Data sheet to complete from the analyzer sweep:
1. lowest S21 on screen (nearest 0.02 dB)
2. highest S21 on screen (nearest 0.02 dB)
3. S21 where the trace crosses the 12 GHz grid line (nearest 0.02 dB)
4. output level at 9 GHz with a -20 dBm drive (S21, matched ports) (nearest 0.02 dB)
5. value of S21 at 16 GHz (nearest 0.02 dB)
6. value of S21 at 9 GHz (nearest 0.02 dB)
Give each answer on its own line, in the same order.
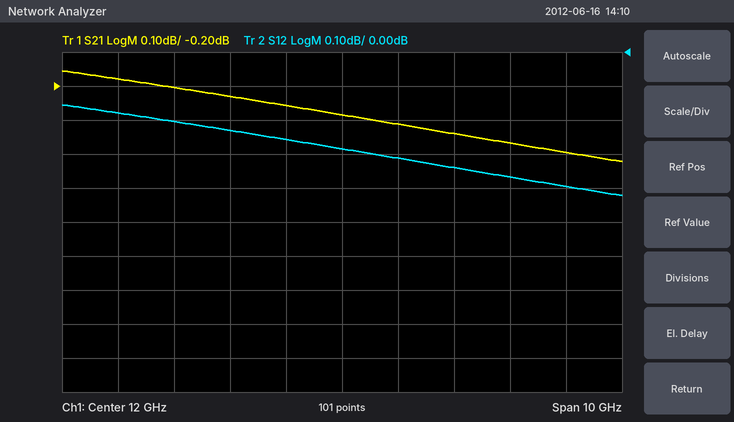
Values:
-0.42 dB
-0.16 dB
-0.28 dB
-20.20 dBm
-0.40 dB
-0.20 dB
